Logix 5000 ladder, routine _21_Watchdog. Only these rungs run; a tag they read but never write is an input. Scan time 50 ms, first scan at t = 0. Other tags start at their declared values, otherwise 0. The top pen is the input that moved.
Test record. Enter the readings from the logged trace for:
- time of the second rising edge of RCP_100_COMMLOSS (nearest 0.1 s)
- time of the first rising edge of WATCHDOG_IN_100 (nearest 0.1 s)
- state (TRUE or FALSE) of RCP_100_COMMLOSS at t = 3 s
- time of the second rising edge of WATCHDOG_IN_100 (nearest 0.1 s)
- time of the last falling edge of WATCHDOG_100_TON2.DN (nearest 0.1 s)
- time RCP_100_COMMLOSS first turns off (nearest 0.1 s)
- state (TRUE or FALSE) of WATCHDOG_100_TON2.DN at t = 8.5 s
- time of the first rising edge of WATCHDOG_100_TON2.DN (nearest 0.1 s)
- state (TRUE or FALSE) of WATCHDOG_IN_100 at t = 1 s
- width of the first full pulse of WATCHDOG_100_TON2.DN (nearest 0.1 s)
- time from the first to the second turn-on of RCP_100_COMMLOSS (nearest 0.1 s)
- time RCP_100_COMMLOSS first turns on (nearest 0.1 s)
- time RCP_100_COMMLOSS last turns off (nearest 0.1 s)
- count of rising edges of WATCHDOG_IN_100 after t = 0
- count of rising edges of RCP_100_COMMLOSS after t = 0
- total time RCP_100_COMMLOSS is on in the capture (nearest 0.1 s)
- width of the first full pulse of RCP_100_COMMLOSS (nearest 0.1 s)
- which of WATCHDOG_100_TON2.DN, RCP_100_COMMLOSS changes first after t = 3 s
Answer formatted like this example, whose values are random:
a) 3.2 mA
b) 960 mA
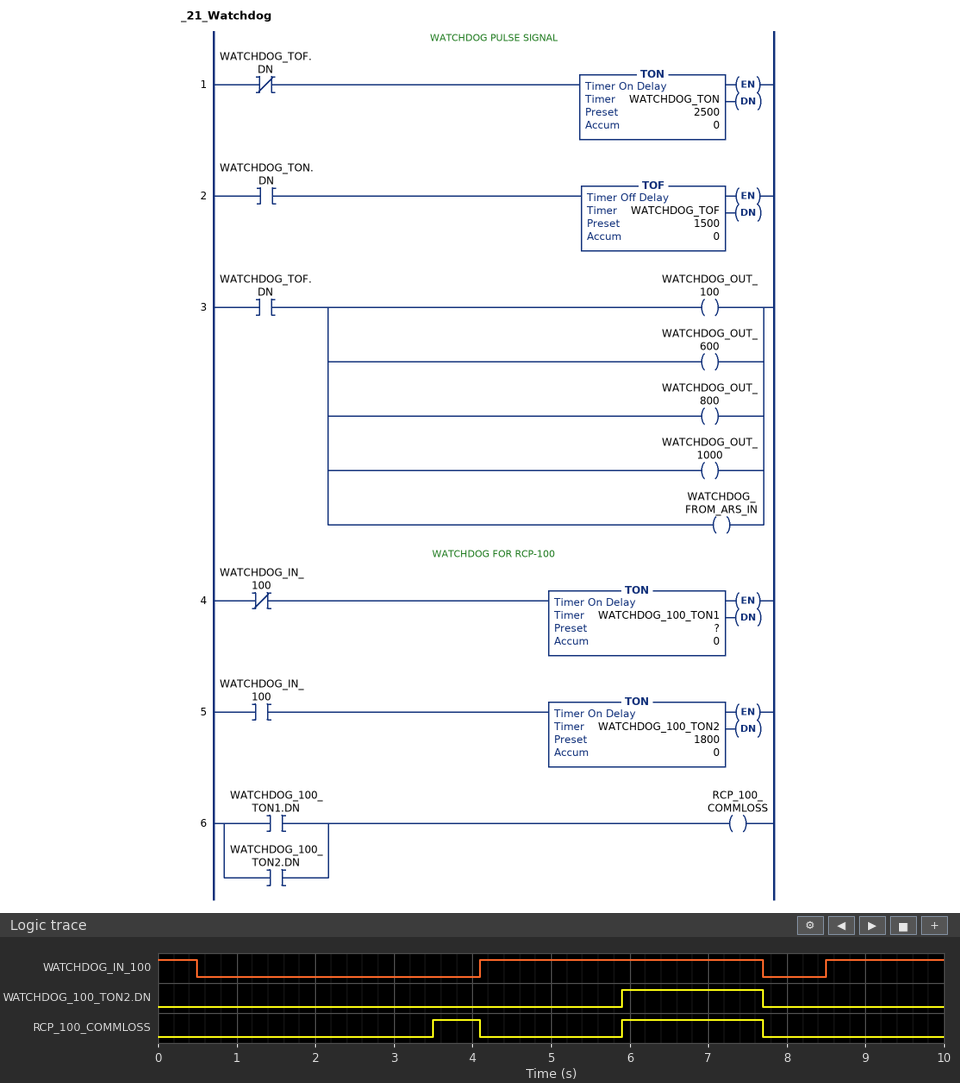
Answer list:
a) 5.9 s
b) 4.1 s
c) FALSE
d) 8.5 s
e) 7.7 s
f) 4.1 s
g) FALSE
h) 5.9 s
i) FALSE
j) 1.8 s
k) 2.4 s
l) 3.5 s
m) 7.7 s
n) 2
o) 2
p) 2.4 s
q) 0.6 s
r) RCP_100_COMMLOSS
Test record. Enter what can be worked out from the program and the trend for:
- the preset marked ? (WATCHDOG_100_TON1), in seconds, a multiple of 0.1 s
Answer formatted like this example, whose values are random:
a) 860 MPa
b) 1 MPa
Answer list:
a) 3.0 s
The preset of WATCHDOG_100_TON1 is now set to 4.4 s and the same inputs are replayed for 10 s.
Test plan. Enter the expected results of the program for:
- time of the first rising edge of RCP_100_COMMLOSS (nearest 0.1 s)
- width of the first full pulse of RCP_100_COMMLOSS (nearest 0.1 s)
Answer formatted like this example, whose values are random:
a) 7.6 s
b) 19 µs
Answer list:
a) 5.9 s
b) 1.8 s
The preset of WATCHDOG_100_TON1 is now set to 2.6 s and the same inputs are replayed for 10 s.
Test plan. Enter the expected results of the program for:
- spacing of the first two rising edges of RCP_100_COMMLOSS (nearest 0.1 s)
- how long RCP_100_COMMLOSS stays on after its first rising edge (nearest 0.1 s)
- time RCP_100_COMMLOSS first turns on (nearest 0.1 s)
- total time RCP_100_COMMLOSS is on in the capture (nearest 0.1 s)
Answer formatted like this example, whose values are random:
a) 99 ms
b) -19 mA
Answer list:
a) 2.8 s
b) 1.0 s
c) 3.1 s
d) 2.8 s
